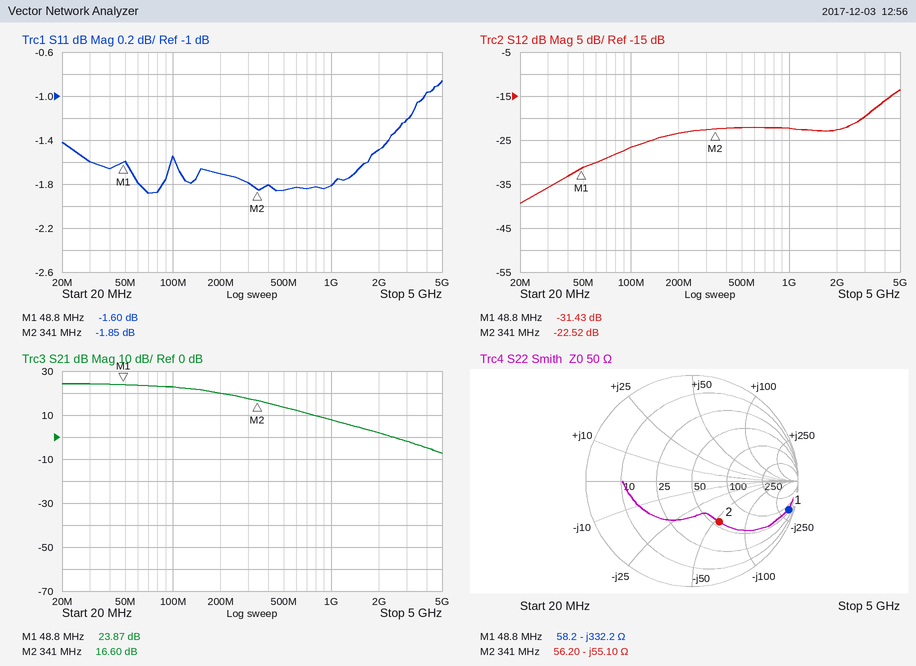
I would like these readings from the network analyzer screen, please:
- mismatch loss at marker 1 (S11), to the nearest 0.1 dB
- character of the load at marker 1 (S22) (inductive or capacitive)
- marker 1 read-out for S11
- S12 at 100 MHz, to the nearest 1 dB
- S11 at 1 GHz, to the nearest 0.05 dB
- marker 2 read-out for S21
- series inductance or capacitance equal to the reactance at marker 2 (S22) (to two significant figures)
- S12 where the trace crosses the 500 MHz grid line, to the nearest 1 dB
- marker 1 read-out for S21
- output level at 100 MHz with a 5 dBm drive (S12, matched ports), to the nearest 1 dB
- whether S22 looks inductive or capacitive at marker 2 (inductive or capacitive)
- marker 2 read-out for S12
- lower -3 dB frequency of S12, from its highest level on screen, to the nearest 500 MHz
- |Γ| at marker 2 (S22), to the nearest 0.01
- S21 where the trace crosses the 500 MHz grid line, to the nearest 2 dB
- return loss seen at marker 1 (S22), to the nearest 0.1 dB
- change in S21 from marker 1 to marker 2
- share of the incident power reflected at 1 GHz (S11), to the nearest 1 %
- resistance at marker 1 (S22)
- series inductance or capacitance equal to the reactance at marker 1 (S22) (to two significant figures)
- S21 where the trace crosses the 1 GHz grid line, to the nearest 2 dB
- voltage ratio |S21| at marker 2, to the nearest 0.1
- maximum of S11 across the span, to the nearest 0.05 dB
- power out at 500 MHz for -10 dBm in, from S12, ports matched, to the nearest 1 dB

5.1 dB
capacitive
-1.60 dB
-27 dB
-1.80 dB
16.60 dB
8.5 pF
-22 dB
23.87 dB
-22 dBm
capacitive
-22.52 dB
4.0 GHz
0.46
14 dB
0.4 dB
-7.27 dB
66 %
58.2 Ω
9.8 pF
8 dB
6.8
-0.85 dB
-32 dBm
